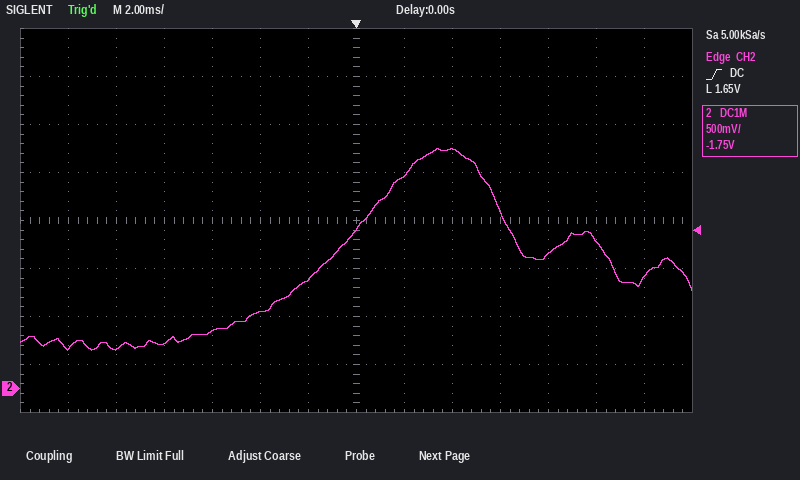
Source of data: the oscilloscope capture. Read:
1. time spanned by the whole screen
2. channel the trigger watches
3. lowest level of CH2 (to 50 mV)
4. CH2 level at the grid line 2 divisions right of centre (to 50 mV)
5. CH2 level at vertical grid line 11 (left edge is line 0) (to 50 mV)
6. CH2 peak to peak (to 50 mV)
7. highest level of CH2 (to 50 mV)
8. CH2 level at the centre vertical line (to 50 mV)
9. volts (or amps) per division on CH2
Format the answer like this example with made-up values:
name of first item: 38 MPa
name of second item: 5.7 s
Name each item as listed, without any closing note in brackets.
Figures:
time spanned by the whole screen: 28 ms
channel the trigger watches: CH2
lowest level of CH2: 400 mV
CH2 level at the grid line 2 divisions right of centre: 2.50 V
CH2 level at vertical grid line 11 (left edge is line 0): 1.40 V
CH2 peak to peak: 2.10 V
highest level of CH2: 2.50 V
CH2 level at the centre vertical line: 1.65 V
volts (or amps) per division on CH2: 500 mV
